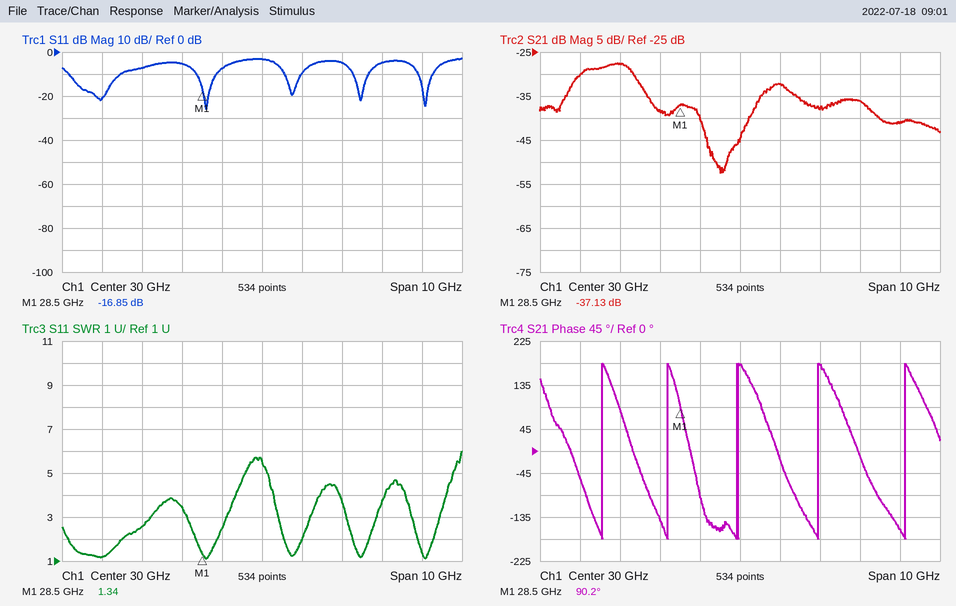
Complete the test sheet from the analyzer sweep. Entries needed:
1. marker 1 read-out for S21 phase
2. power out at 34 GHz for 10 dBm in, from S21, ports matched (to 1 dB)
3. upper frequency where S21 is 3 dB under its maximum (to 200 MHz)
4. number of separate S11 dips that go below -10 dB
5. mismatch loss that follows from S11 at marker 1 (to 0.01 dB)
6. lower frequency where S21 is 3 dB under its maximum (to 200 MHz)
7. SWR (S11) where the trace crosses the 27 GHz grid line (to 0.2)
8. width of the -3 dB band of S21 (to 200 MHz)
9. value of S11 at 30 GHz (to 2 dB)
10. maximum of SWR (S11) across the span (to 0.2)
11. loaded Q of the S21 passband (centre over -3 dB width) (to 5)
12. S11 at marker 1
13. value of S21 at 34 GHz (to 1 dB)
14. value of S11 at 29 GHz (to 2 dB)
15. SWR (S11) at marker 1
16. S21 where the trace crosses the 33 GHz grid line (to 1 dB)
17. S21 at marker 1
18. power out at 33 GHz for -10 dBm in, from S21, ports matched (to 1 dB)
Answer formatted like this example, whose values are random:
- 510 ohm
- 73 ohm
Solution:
- 90.2°
- -31 dBm
- 27.4 GHz
- 5
- 0.09 dB
- 26.0 GHz
- 2.6
- 1.4 GHz
- -4 dB
- 6.0
- 20
- -16.85 dB
- -41 dB
- -8 dB
- 1.34
- -36 dB
- -37.13 dB
- -46 dBm
